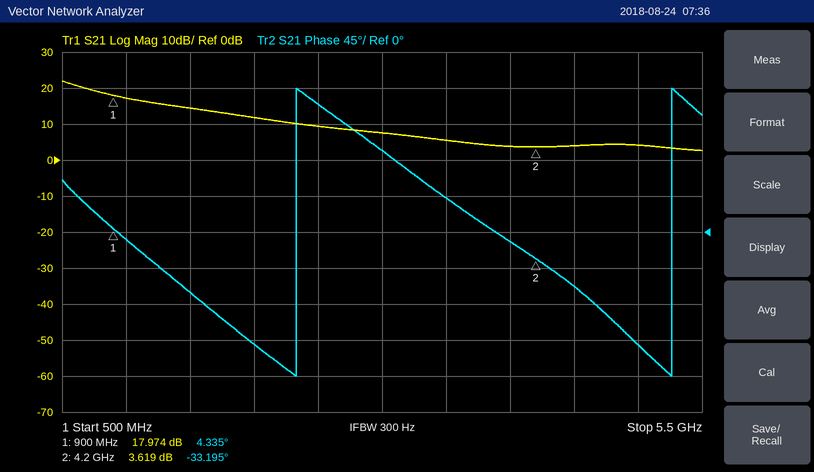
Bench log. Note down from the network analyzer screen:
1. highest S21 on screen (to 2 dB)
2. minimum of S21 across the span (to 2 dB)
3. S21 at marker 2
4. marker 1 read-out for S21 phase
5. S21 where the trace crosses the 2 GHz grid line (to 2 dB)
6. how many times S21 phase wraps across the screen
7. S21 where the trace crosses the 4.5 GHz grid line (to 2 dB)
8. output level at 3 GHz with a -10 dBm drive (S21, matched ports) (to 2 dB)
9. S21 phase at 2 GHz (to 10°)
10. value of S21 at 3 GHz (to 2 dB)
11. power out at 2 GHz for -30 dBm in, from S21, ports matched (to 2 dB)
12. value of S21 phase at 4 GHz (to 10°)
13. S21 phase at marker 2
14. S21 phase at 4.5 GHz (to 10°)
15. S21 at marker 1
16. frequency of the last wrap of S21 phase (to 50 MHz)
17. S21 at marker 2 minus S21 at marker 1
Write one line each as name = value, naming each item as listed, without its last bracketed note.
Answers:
highest S21 on screen = 22 dB
minimum of S21 across the span = 2 dB
S21 at marker 2 = 3.619 dB
marker 1 read-out for S21 phase = 4.335°
S21 where the trace crosses the 2 GHz grid line = 12 dB
how many times S21 phase wraps across the screen = 2
S21 where the trace crosses the 4.5 GHz grid line = 4 dB
output level at 3 GHz with a -10 dBm drive (S21, matched ports) = -2 dBm
S21 phase at 2 GHz = -140°
value of S21 at 3 GHz = 8 dB
power out at 2 GHz for -30 dBm in, from S21, ports matched = -18 dBm
value of S21 phase at 4 GHz = -10°
S21 phase at marker 2 = -33.195°
S21 phase at 4.5 GHz = -70°
S21 at marker 1 = 17.974 dB
frequency of the last wrap of S21 phase = 5.25 GHz
S21 at marker 2 minus S21 at marker 1 = -14.355 dB
